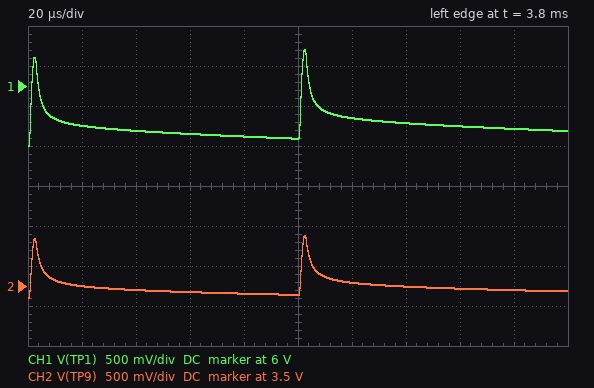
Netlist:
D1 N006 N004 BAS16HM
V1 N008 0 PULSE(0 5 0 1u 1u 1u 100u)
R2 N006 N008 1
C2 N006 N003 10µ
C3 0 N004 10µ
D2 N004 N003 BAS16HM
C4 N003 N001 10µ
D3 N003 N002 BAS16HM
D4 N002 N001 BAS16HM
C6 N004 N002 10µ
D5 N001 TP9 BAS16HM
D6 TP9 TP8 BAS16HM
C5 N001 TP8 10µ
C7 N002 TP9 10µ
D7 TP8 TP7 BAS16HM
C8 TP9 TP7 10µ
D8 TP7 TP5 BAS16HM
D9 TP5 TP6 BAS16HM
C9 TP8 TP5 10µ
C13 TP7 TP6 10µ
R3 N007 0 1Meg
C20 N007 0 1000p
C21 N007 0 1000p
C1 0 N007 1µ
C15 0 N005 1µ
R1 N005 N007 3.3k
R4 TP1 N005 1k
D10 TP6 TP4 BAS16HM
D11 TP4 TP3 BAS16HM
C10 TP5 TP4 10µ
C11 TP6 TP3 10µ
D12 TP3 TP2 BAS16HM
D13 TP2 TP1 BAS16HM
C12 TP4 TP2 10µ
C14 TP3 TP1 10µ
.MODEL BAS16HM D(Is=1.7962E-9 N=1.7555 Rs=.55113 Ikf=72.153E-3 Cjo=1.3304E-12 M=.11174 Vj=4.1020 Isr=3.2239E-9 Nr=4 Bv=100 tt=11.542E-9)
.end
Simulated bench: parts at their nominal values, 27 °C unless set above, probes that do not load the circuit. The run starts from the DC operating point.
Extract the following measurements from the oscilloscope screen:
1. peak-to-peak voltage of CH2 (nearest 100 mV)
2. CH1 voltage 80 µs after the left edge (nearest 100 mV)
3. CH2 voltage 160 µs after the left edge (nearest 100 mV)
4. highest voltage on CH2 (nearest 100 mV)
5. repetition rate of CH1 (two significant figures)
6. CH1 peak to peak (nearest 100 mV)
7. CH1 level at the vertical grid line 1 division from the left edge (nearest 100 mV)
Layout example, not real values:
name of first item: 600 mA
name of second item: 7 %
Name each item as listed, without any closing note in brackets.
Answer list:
peak-to-peak voltage of CH2: 800 mV
CH1 voltage 80 µs after the left edge: 5.4 V
CH2 voltage 160 µs after the left edge: 3.5 V
highest voltage on CH2: 4.1 V
repetition rate of CH1: 10 kHz
CH1 peak to peak: 1.2 V
CH1 level at the vertical grid line 1 division from the left edge: 5.5 V
